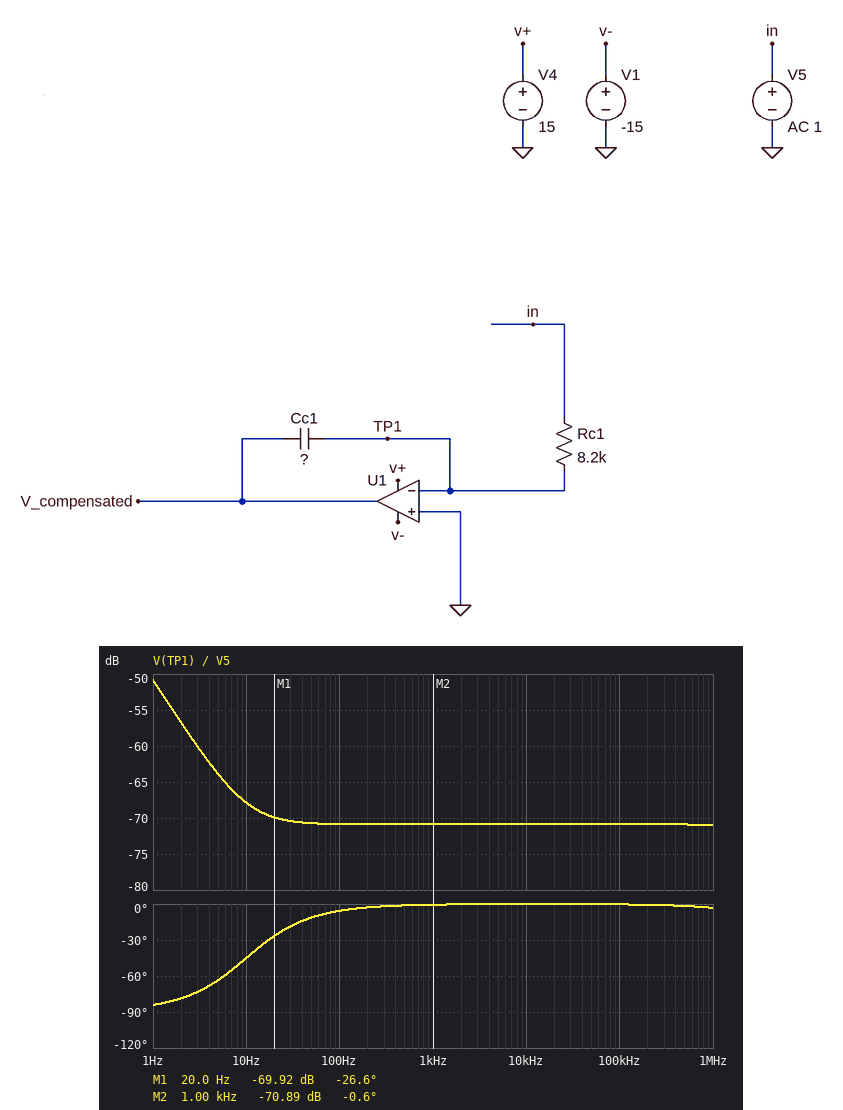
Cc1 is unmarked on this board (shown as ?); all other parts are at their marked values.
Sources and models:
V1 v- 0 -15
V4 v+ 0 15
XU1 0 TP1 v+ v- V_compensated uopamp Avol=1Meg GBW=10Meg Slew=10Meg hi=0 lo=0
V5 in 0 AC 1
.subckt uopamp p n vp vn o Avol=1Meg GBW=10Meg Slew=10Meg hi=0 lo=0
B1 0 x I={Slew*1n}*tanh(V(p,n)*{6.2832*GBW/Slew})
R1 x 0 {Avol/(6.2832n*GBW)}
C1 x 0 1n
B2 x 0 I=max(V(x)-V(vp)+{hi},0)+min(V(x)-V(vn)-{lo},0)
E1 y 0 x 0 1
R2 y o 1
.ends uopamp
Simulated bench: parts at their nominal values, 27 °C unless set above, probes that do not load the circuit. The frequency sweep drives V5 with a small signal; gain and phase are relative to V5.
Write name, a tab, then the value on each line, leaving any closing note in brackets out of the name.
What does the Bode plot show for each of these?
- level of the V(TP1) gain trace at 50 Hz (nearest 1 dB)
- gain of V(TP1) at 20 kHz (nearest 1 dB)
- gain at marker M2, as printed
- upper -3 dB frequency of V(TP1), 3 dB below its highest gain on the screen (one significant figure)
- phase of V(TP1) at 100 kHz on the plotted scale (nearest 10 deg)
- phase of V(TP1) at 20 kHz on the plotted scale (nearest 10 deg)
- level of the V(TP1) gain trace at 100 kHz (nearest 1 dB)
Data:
level of the V(TP1) gain trace at 50 Hz	-71 dB
gain of V(TP1) at 20 kHz	-71 dB
gain at marker M2, as printed	-70.89 dB
upper -3 dB frequency of V(TP1), 3 dB below its highest gain on the screen	1 Hz
phase of V(TP1) at 100 kHz on the plotted scale	0 deg
phase of V(TP1) at 20 kHz on the plotted scale	0 deg
level of the V(TP1) gain trace at 100 kHz	-71 dB
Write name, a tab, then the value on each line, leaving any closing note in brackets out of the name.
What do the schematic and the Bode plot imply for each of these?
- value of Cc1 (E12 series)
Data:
value of Cc1	6.8 nF
